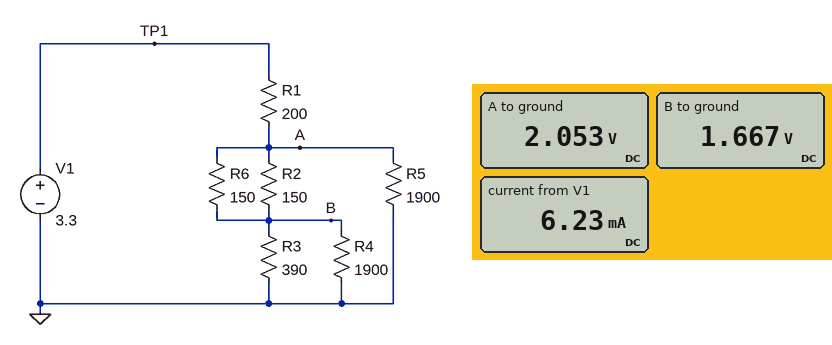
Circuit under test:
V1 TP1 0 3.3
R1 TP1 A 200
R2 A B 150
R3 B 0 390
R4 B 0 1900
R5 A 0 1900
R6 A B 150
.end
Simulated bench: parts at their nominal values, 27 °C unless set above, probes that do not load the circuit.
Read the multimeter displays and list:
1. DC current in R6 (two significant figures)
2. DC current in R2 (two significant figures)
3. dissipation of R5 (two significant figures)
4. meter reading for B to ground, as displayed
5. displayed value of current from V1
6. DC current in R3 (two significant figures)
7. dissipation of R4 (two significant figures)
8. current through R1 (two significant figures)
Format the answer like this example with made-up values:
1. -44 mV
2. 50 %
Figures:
1. 2.6 mA
2. 2.6 mA
3. 2.2 mW
4. 1.667 V
5. 6.23 mA
6. 4.3 mA
7. 1.5 mW
8. 6.2 mA
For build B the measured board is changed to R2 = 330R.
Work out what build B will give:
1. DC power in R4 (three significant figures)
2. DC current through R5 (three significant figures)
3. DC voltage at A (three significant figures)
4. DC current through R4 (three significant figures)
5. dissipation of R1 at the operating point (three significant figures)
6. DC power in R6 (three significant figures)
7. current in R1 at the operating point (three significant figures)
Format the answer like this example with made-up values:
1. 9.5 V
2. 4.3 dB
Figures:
1. 1.33 mW
2. 1.10 mA
3. 2.10 V
4. 837 µA
5. 7.24 mW
6. 1.71 mW
7. 6.02 mA
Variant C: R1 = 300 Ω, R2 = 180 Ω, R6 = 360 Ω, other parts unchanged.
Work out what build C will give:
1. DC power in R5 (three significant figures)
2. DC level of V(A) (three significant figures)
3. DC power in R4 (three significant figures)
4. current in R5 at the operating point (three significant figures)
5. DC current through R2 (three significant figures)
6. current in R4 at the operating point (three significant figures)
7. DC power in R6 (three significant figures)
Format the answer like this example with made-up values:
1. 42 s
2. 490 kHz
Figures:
1. 1.70 mW
2. 1.80 V
3. 907 µW
4. 947 µA
5. 2.70 mA
6. 691 µA
7. 658 µW
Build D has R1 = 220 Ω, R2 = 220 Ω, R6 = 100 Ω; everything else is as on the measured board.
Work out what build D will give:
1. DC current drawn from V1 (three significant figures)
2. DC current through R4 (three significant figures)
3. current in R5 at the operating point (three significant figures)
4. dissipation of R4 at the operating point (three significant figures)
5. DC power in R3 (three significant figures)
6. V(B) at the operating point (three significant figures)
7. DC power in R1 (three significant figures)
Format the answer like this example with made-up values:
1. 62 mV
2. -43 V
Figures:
1. 6.05 mA
2. 854 µA
3. 1.04 mA
4. 1.39 mW
5. 6.76 mW
6. 1.62 V
7. 8.06 mW
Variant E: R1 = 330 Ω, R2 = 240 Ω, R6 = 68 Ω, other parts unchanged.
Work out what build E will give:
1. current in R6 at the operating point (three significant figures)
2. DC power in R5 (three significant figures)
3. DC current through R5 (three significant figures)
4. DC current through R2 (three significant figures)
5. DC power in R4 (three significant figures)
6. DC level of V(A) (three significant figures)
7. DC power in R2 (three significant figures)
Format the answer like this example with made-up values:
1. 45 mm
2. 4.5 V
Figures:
1. 3.33 mA
2. 1.36 mW
3. 847 µA
4. 944 µA
5. 1.01 mW
6. 1.61 V
7. 214 µW
